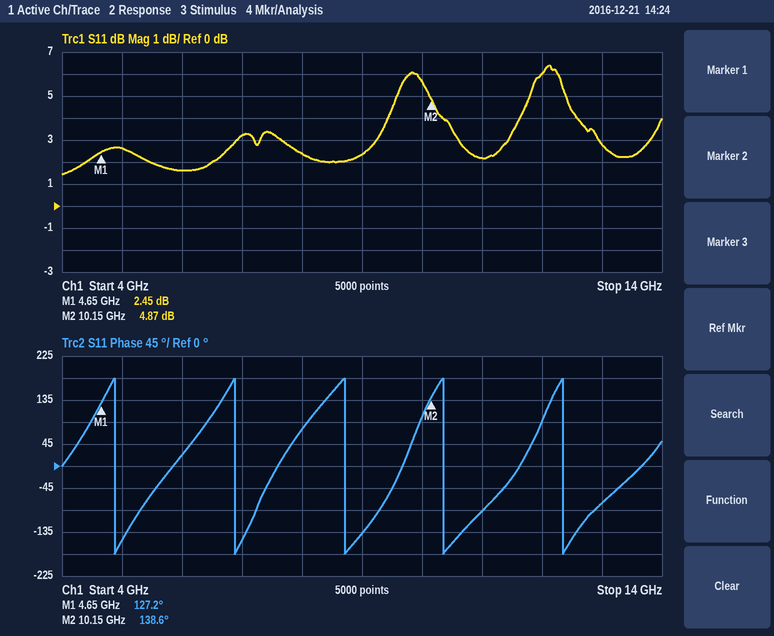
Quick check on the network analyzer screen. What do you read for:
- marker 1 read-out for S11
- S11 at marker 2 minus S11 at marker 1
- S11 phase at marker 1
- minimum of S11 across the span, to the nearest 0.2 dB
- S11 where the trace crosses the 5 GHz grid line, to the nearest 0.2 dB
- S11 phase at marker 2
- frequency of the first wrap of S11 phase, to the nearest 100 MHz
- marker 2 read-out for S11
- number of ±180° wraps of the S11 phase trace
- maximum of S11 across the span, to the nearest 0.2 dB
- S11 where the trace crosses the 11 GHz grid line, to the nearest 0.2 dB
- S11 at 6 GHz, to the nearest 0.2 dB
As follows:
2.45 dB
2.42 dB
127.2°
1.4 dB
2.6 dB
138.6°
4.9 GHz
4.87 dB
5
6.4 dB
2.2 dB
1.6 dB
